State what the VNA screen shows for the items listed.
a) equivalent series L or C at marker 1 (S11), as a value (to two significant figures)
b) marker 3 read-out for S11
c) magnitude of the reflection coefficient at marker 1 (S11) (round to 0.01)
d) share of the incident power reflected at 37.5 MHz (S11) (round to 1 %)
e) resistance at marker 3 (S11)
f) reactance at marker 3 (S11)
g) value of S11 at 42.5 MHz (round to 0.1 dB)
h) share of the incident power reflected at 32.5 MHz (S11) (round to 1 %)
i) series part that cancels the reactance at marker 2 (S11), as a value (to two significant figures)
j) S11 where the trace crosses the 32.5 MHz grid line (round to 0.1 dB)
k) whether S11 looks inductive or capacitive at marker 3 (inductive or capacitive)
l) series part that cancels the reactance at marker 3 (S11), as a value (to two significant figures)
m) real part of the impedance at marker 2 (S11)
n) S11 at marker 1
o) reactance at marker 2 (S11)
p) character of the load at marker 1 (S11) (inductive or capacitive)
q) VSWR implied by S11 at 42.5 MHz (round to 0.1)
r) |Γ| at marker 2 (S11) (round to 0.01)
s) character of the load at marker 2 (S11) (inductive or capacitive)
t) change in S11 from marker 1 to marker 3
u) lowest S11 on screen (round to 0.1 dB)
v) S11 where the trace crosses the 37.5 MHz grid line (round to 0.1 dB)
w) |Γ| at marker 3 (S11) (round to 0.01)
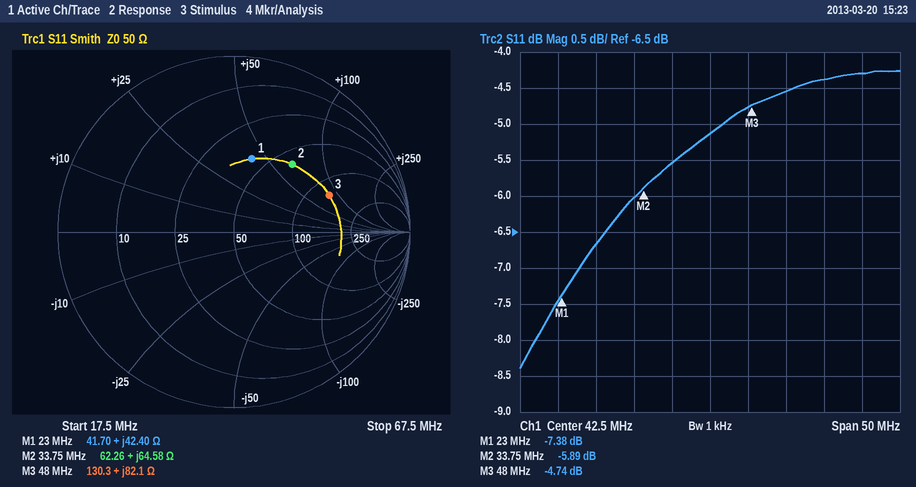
290 nH
-4.74 dB
0.43
28 %
130.3 Ω
+82.1 Ω
-5.1 dB
25 %
73 pF
-6.0 dB
inductive
40 pF
62.26 Ω
-7.38 dB
+64.58 Ω
inductive
3.5
0.51
inductive
2.64 dB
-8.4 dB
-5.5 dB
0.58
